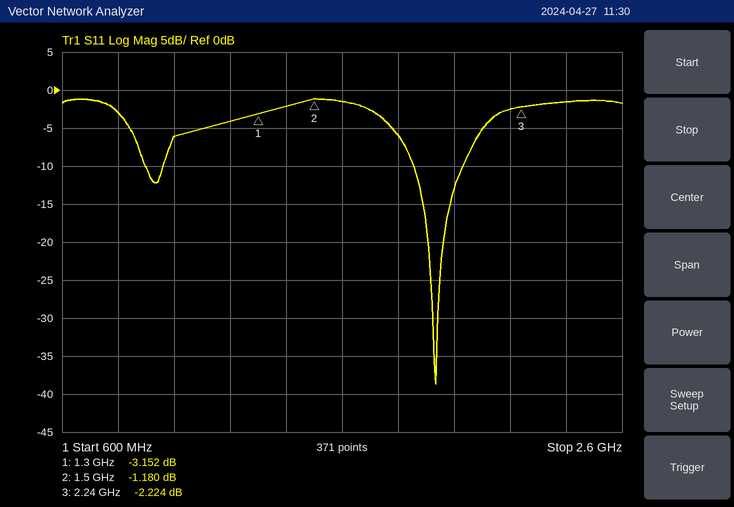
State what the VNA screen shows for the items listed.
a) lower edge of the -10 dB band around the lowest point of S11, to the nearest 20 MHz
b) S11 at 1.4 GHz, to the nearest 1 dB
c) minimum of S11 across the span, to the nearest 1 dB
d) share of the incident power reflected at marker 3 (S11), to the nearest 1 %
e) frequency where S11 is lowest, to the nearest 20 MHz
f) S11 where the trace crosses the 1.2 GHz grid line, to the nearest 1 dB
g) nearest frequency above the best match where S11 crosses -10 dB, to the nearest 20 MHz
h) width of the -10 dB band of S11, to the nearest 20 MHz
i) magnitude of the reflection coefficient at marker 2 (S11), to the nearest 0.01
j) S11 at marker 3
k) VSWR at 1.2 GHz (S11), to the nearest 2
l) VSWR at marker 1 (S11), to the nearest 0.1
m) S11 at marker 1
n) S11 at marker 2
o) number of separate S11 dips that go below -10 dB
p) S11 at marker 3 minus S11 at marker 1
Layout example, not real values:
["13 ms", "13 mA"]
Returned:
["1.86 GHz", "-2 dB", "-39 dB", "60 %", "1.94 GHz", "-4 dB", "2.04 GHz", "180 MHz", "0.87", "-2.224 dB", "4", "5.6", "-3.152 dB", "-1.180 dB", "2", "0.928 dB"]
